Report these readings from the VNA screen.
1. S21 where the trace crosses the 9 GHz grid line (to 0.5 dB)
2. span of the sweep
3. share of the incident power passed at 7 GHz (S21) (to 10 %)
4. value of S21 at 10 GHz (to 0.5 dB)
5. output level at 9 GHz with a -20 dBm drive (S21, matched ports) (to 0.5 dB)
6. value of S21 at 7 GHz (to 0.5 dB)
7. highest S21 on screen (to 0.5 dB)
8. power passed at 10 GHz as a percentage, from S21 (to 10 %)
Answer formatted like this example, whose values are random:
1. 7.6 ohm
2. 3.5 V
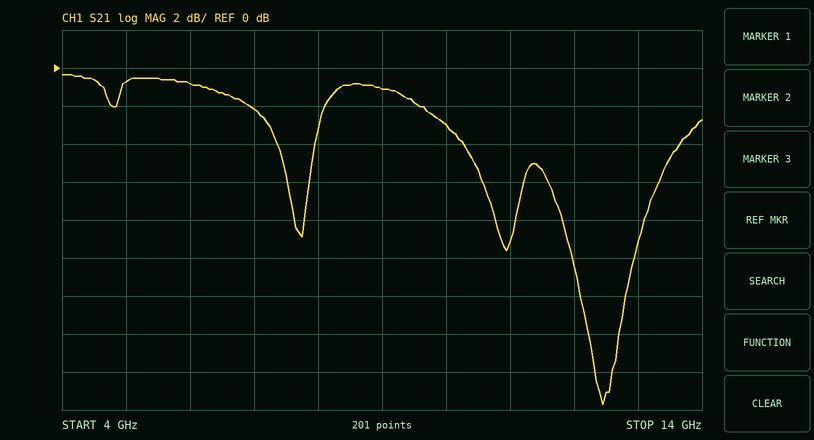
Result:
1. -1.0 dB
2. 10 GHz
3. 60 %
4. -3.0 dB
5. -21.0 dBm
6. -2.0 dB
7. -0.5 dB
8. 50 %
